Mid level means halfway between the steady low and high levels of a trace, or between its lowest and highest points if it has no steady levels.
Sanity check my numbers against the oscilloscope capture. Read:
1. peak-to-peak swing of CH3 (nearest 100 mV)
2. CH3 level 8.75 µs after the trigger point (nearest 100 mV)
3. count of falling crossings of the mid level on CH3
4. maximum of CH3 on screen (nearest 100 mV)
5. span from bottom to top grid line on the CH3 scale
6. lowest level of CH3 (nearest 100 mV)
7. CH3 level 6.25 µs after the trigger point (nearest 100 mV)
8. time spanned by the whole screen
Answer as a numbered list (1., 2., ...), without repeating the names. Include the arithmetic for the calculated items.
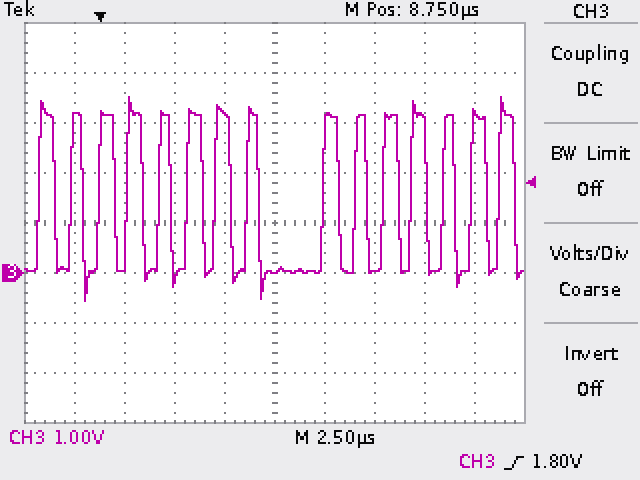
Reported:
1. 3.5 V − (-600 mV) = 4.1 V
2. 0.0 V
3. 15
4. 3.5 V
5. 8 V
6. -600 mV
7. 3.2 V
8. 25 µs
